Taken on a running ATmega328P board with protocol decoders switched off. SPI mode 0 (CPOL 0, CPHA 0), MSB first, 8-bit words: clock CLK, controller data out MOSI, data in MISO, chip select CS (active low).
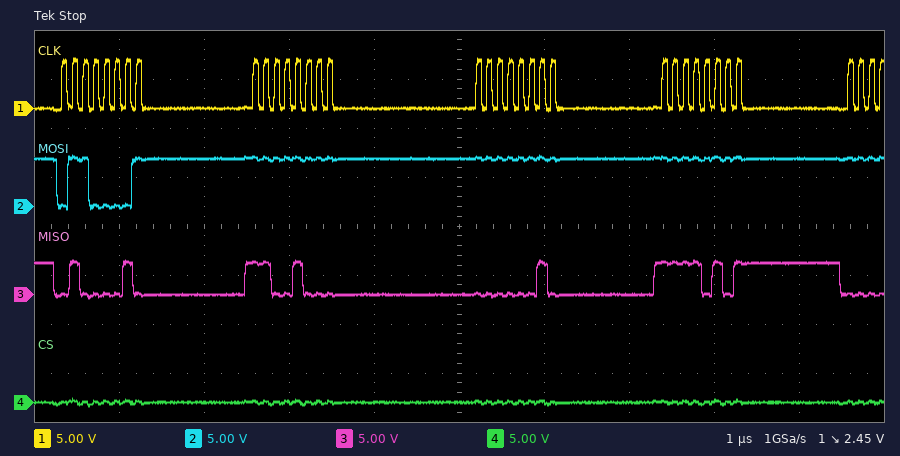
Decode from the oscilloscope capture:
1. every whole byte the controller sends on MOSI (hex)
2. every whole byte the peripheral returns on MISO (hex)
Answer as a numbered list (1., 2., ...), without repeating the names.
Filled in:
1. 61 FF FF FF
2. 42 C8 02 F5
